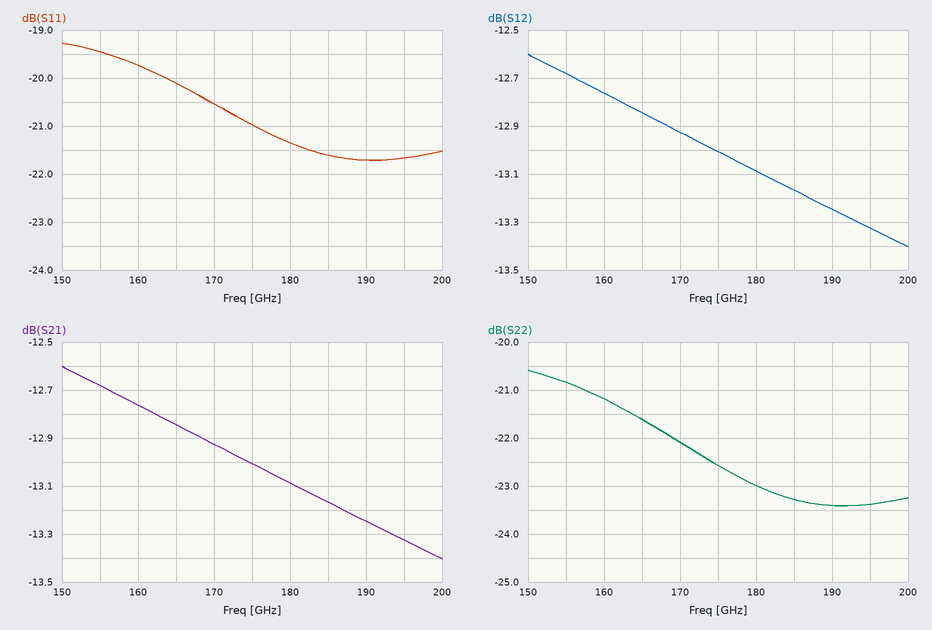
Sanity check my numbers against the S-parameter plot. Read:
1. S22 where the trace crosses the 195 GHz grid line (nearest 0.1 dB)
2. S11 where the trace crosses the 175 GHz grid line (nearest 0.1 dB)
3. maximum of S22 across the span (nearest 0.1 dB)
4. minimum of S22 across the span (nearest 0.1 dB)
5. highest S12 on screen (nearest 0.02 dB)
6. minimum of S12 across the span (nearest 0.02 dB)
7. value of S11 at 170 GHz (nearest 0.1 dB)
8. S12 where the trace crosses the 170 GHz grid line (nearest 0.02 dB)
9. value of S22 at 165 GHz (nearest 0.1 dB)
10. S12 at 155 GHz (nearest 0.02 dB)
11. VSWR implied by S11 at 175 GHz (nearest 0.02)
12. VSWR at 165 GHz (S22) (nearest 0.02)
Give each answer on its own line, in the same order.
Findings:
-23.4 dB
-21.0 dB
-20.6 dB
-23.4 dB
-12.60 dB
-13.40 dB
-20.5 dB
-12.92 dB
-21.6 dB
-12.68 dB
1.20
1.18
